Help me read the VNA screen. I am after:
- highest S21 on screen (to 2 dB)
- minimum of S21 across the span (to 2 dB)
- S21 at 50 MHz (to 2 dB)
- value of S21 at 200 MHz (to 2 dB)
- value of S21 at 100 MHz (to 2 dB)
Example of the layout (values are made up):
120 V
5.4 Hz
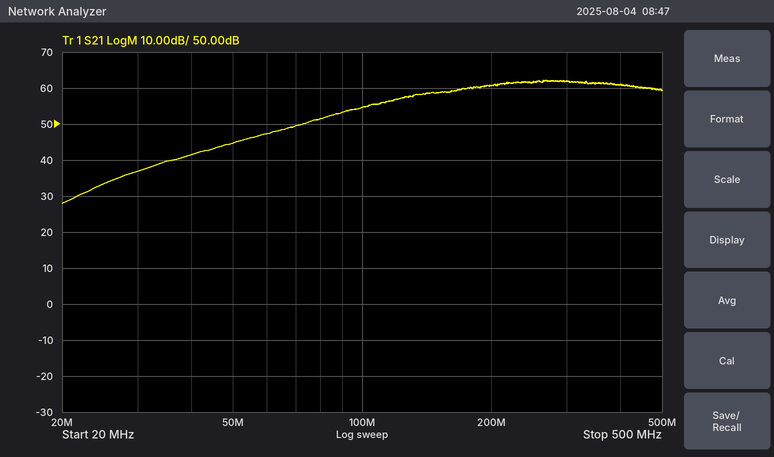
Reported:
62 dB
28 dB
44 dB
60 dB
54 dB
